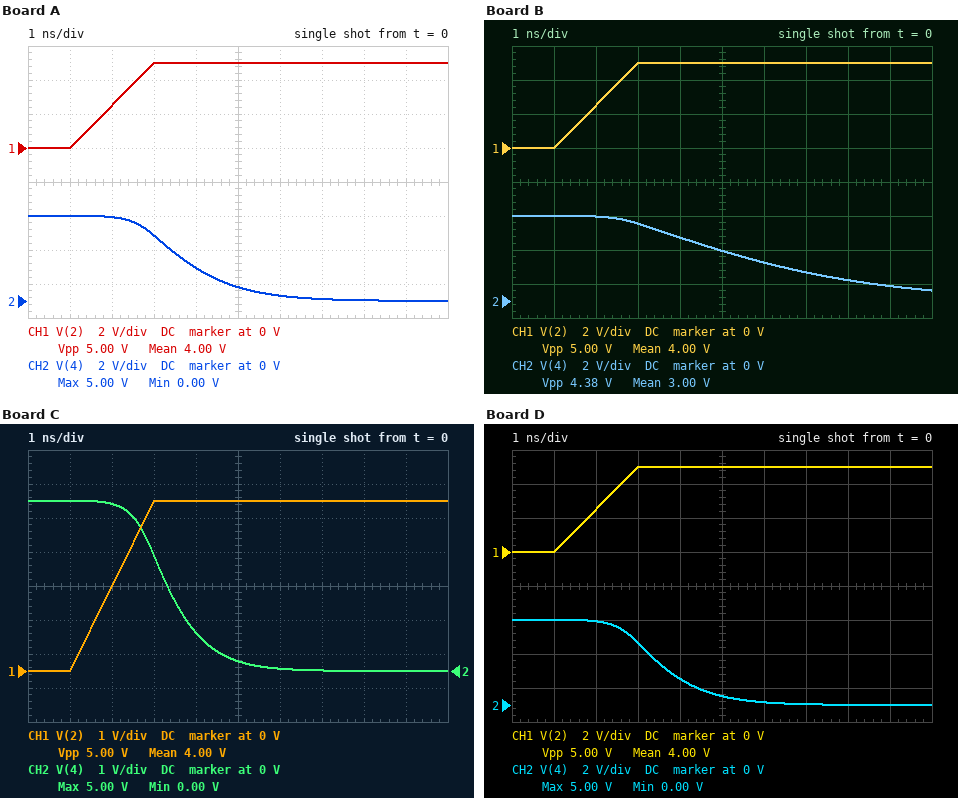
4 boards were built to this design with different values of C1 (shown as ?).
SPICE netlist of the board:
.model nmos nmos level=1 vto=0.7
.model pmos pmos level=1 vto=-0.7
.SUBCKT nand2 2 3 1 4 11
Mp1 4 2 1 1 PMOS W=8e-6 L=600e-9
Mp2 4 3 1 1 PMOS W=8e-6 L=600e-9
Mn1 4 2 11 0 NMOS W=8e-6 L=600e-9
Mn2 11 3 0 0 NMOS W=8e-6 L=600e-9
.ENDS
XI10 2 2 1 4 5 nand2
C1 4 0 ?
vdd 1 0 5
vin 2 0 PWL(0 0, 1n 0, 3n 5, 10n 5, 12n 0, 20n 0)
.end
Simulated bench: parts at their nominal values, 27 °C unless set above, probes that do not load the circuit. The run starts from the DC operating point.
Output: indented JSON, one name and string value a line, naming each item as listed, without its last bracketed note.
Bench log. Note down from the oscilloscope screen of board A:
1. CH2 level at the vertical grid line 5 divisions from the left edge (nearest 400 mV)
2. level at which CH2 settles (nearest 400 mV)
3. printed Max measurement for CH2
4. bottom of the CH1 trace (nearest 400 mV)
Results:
{
  "CH2 level at the vertical grid line 5 divisions from the left edge": "800 mV",
  "level at which CH2 settles": "0 V",
  "printed Max measurement for CH2": "5.00 V",
  "bottom of the CH1 trace": "0 V"
}
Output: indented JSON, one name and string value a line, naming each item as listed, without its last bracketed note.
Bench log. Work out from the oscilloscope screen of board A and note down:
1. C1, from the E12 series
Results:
{
  "C1, from the E12 series": "560 fF"
}
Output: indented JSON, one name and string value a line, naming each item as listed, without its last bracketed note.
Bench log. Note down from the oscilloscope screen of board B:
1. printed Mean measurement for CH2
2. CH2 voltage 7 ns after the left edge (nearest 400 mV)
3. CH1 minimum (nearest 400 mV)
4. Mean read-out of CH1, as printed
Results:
{
  "printed Mean measurement for CH2": "3.00 V",
  "CH2 voltage 7 ns after the left edge": "1.6 V",
  "CH1 minimum": "0 V",
  "Mean read-out of CH1, as printed": "4.00 V"
}
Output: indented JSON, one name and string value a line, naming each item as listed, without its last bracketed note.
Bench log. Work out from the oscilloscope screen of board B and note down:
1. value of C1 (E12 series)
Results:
{
  "value of C1": "1.5 pF"
}
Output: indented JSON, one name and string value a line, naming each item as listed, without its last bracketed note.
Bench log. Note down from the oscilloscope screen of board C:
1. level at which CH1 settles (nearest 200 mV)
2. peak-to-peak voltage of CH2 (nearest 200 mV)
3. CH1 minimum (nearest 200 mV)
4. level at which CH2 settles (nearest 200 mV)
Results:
{
  "level at which CH1 settles": "5.0 V",
  "peak-to-peak voltage of CH2": "5.0 V",
  "CH1 minimum": "0 V",
  "level at which CH2 settles": "0 V"
}
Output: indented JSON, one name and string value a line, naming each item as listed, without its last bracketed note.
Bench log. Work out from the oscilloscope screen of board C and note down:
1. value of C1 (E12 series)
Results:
{
  "value of C1": "390 fF"
}
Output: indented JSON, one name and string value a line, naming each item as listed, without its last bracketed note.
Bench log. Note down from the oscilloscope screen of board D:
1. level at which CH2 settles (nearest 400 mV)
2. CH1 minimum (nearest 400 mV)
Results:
{
  "level at which CH2 settles": "0 V",
  "CH1 minimum": "0 V"
}
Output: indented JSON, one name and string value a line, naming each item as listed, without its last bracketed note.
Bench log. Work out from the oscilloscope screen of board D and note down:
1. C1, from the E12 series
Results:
{
  "C1, from the E12 series": "470 fF"
}
